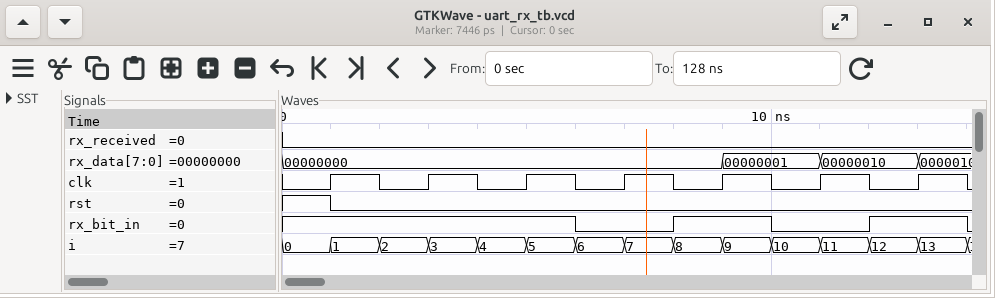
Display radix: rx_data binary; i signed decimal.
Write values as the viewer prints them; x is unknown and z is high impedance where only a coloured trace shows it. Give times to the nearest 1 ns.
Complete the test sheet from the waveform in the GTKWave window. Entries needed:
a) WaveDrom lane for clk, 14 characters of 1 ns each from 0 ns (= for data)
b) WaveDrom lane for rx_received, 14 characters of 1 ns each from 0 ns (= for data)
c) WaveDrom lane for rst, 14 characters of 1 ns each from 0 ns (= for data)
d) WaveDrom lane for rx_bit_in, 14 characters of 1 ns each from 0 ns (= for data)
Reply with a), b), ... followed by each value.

a) {name: 'clk', wave: '01010101010101'}
b) {name: 'rx_received', wave: '0.............'}
c) {name: 'rst', wave: '10............'}
d) {name: 'rx_bit_in', wave: '1.....0.1.0.1.'}
